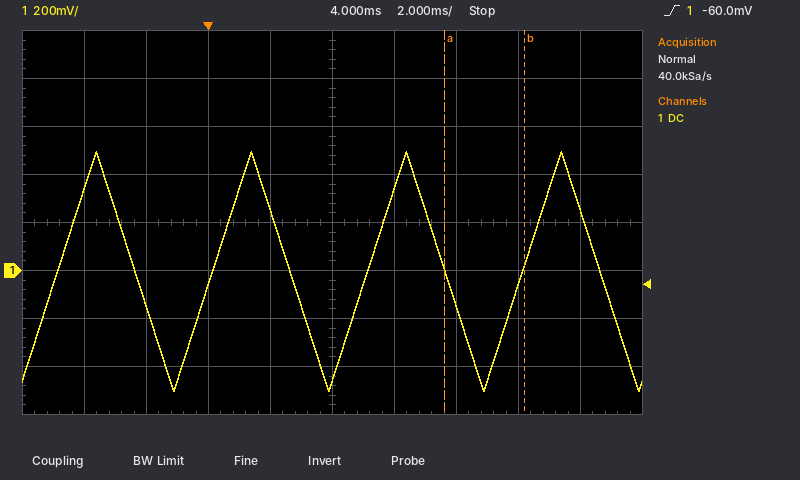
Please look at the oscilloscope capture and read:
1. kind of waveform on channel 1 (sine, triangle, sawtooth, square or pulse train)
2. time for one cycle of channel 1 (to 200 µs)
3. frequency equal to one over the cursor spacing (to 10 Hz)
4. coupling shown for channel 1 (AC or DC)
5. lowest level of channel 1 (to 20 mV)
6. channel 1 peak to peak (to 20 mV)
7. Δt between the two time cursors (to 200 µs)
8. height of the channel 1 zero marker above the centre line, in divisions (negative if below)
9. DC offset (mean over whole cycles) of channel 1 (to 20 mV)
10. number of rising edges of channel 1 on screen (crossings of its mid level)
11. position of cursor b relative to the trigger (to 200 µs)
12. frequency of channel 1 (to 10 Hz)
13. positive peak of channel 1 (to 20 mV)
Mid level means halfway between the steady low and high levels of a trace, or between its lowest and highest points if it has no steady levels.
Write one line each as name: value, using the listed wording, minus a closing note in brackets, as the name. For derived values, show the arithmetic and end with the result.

kind of waveform on channel 1: triangle
time for one cycle of channel 1: 5.0 ms
frequency equal to one over the cursor spacing: 1 / 2.6 ms ≈ 380 Hz
coupling shown for channel 1: DC
lowest level of channel 1: -500 mV
channel 1 peak to peak: 500 mV − (-500 mV) = 1.00 V
Δt between the two time cursors: 2.6 ms
height of the channel 1 zero marker above the centre line, in divisions: -1.0 div
DC offset (mean over whole cycles) of channel 1: (500 mV + (-500 mV)) / 2 ≈ 0 mV
number of rising edges of channel 1 on screen: 4
position of cursor b relative to the trigger: +10.2 ms
frequency of channel 1: 1 / 5.0 ms ≈ 200 Hz
positive peak of channel 1: 500 mV
